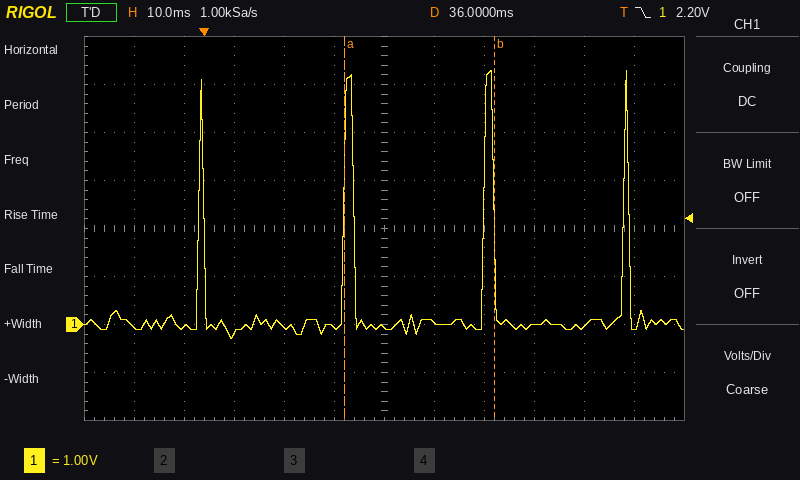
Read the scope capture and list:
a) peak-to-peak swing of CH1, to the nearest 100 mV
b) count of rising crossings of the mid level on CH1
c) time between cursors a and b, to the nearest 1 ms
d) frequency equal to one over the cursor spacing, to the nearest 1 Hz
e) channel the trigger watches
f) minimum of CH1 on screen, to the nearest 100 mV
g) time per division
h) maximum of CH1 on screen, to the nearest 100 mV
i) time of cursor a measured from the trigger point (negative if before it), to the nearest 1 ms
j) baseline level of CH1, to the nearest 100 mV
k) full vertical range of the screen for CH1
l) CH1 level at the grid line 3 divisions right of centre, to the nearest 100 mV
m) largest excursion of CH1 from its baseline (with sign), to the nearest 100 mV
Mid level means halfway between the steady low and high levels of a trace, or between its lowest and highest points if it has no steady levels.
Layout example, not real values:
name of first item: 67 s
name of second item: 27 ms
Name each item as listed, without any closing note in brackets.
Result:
peak-to-peak swing of CH1, to the nearest 100 mV: 5.6 V
count of rising crossings of the mid level on CH1: 4
time between cursors a and b, to the nearest 1 ms: 30 ms
frequency equal to one over the cursor spacing, to the nearest 1 Hz: 33 Hz
channel the trigger watches: CH1
minimum of CH1 on screen, to the nearest 100 mV: -300 mV
time per division: 10 ms
maximum of CH1 on screen, to the nearest 100 mV: 5.3 V
time of cursor a measured from the trigger point (negative if before it), to the nearest 1 ms: +28 ms
baseline level of CH1, to the nearest 100 mV: 0.0 V
full vertical range of the screen for CH1: 8 V
CH1 level at the grid line 3 divisions right of centre, to the nearest 100 mV: 0.0 V
largest excursion of CH1 from its baseline (with sign), to the nearest 100 mV: +5.3 V
